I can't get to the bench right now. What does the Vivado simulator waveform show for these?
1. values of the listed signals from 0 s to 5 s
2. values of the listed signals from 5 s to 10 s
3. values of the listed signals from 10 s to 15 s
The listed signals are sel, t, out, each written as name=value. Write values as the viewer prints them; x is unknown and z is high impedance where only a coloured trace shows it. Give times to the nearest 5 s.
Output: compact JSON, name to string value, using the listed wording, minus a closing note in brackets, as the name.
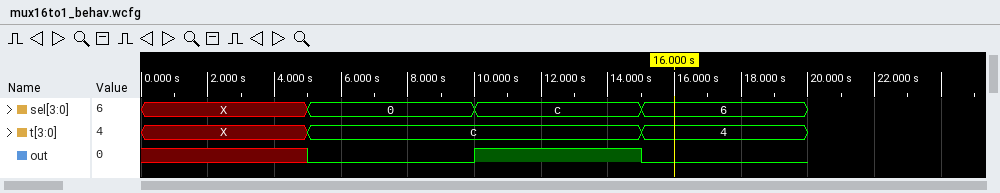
{"values of the listed signals from 0 s to 5 s": "sel=X, t=X, out=x", "values of the listed signals from 5 s to 10 s": "sel=0, t=c, out=0", "values of the listed signals from 10 s to 15 s": "sel=c, t=c, out=1"}
